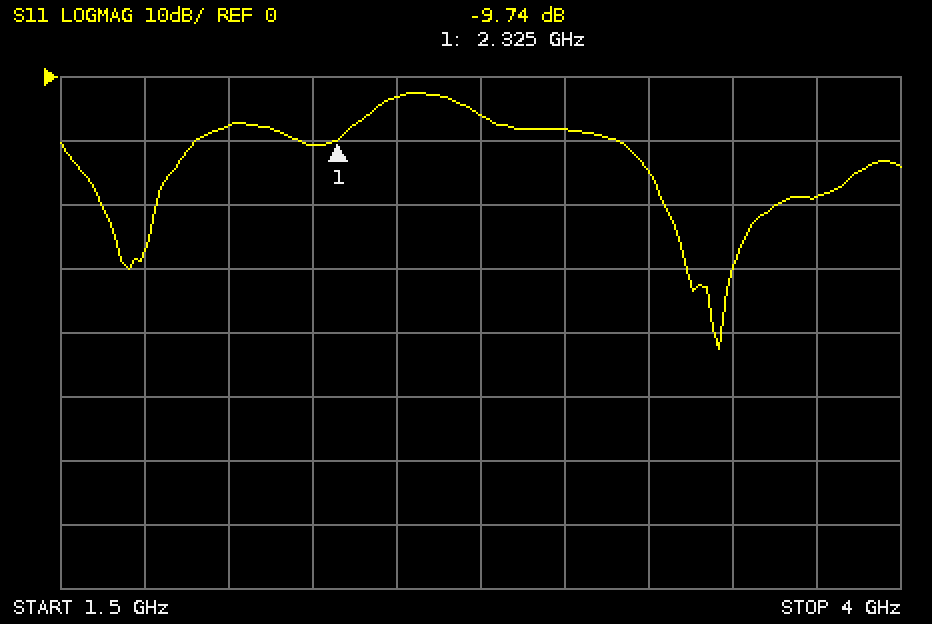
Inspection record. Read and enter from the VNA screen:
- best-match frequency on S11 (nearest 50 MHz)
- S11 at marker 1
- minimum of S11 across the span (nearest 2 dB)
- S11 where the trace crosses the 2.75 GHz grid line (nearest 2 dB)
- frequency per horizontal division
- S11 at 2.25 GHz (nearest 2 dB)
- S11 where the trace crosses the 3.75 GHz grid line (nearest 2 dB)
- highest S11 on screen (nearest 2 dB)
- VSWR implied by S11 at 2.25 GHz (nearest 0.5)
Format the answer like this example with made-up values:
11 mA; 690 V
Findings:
3.45 GHz; -9.74 dB; -42 dB; -6 dB; 250 MHz; -10 dB; -18 dB; -2 dB; 2.0
